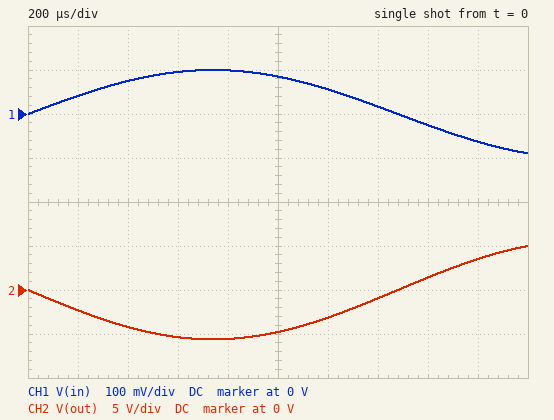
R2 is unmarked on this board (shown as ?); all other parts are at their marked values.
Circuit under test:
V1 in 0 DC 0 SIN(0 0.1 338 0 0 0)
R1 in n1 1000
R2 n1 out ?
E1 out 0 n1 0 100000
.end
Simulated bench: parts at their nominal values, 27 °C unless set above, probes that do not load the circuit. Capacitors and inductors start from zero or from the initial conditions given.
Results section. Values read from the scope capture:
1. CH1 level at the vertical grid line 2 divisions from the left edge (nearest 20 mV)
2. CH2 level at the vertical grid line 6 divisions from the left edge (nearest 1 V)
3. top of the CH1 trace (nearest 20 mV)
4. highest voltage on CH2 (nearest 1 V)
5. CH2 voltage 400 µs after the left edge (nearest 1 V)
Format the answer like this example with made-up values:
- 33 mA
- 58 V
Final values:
- 80 mV
- -3 V
- 100 mV
- 5 V
- -4 V
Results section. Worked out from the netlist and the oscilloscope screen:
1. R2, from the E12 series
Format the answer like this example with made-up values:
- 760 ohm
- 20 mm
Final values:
- 56 kΩ
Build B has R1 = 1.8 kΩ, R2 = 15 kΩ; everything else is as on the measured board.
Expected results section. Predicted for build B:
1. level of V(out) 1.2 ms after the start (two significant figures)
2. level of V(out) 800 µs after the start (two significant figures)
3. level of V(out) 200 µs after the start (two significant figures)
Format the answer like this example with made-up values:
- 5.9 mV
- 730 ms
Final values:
- -470 mV
- -830 mV
- -340 mV
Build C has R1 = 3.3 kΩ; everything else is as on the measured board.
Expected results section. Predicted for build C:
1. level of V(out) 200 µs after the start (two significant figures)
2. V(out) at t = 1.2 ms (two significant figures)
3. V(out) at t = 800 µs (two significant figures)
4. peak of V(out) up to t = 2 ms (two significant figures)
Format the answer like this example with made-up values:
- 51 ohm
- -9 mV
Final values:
- -700 mV
- -950 mV
- -1.7 V
- 1.5 V
